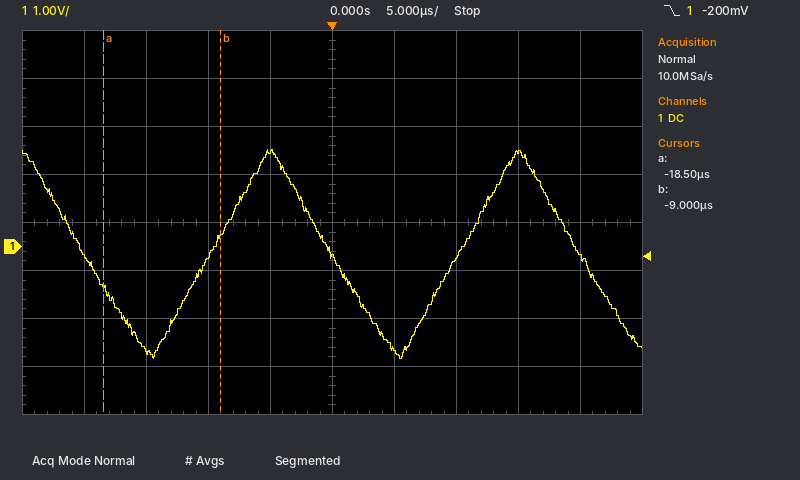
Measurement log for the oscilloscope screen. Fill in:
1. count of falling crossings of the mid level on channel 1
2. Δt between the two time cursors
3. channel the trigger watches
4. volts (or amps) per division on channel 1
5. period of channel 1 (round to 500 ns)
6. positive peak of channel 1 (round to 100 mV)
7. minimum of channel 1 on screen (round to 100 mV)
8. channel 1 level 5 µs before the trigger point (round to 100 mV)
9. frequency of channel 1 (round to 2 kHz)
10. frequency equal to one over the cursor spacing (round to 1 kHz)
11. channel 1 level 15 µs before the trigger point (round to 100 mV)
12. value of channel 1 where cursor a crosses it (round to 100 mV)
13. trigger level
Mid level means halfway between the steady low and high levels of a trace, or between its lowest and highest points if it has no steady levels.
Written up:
3
9.5 µs
channel 1
1 V
20.0 µs
2.0 V
-2.3 V
2.0 V
50 kHz
105 kHz
-2.2 V
-900 mV
-200 mV
